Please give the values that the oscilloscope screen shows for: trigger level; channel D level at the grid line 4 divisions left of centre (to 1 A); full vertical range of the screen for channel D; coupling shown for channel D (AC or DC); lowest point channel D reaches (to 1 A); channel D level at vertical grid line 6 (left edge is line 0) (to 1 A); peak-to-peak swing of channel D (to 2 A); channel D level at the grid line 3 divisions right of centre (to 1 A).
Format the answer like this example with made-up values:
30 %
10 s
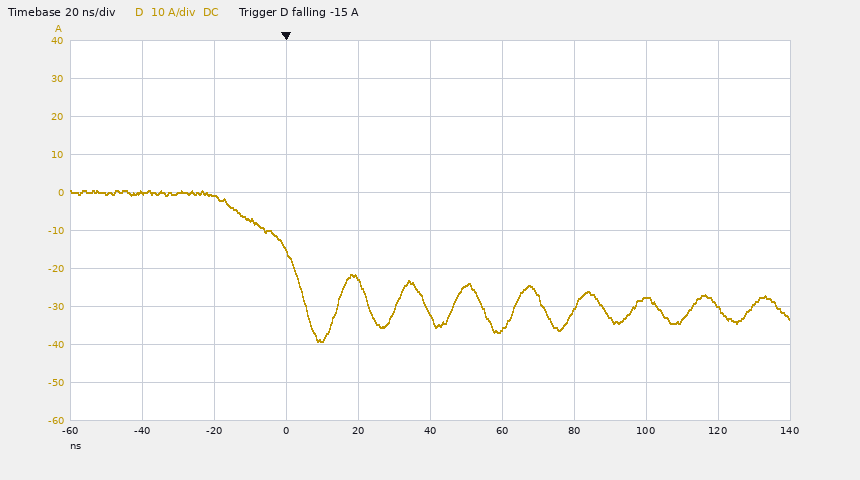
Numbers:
-15 A
0 A
100 A
DC
-39 A
-36 A
40 A
-28 A
